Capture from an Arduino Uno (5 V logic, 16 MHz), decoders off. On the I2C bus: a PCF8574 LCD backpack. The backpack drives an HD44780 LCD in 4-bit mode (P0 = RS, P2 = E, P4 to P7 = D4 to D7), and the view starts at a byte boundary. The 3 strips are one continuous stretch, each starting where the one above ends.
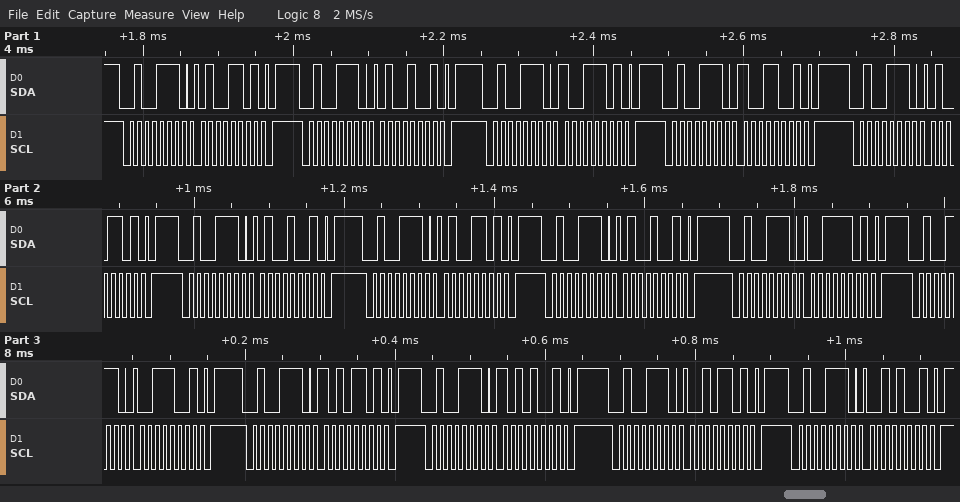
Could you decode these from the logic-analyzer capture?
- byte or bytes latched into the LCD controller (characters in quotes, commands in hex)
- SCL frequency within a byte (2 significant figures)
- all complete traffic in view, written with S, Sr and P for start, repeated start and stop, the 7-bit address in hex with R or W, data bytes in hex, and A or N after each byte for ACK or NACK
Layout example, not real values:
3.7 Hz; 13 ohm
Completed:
'I' 'D' ':'; 100 kHz; S 27W A 4D A P S 27W A 49 A P S 27W A 9D A P S 27W A 99 A P S 27W A 4D A P S 27W A 49 A P S 27W A 4D A P S 27W A 49 A P S 27W A 3D A P S 27W A 39 A P S 27W A AD A P S 27W A A9 A P S 27W A 2D A P S 27W A 29 A P
